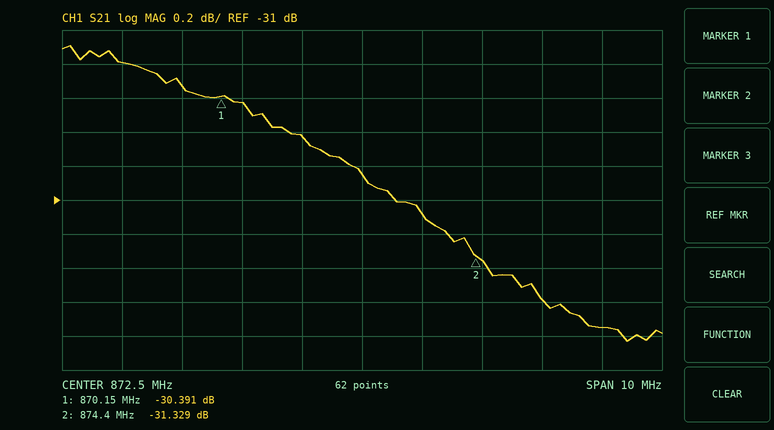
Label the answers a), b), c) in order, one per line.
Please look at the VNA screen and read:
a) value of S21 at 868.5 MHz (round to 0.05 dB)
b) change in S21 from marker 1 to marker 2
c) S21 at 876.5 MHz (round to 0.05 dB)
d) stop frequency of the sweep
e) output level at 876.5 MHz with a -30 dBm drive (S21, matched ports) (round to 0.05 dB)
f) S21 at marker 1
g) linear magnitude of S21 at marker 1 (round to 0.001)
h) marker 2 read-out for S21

a) -30.20 dB
b) -0.938 dB
c) -31.75 dB
d) 877.5 MHz
e) -61.75 dBm
f) -30.391 dB
g) 0.030
h) -31.329 dB
